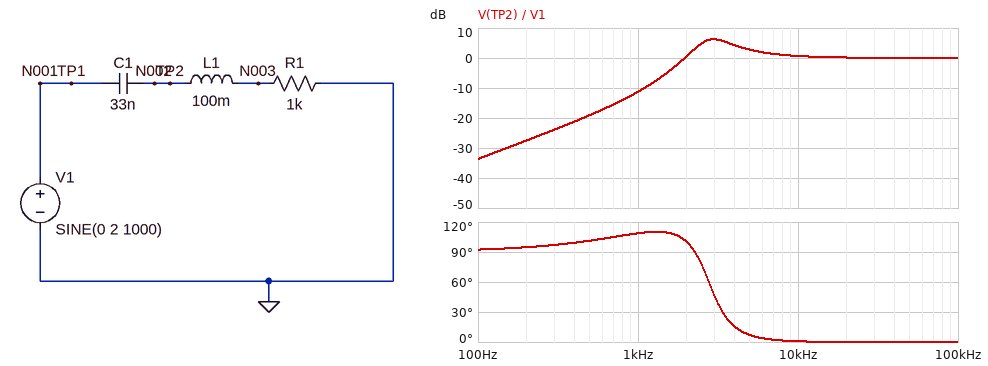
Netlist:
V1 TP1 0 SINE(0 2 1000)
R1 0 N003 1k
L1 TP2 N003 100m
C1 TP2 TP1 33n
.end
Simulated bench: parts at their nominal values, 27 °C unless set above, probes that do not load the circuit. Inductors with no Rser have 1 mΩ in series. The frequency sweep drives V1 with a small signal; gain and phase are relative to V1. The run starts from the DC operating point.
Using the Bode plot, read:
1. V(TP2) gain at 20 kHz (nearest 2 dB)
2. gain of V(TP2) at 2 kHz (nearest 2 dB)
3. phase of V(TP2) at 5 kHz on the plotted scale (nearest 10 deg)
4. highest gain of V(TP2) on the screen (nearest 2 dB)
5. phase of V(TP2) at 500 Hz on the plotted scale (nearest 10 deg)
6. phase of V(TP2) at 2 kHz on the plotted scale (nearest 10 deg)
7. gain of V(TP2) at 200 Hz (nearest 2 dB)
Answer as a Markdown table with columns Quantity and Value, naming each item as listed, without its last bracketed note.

| Quantity | Value |
|---|---|
| V(TP2) gain at 20 kHz | 0 dB |
| gain of V(TP2) at 2 kHz | 0 dB |
| phase of V(TP2) at 5 kHz on the plotted scale | 10 deg |
| highest gain of V(TP2) on the screen | 6 dB |
| phase of V(TP2) at 500 Hz on the plotted scale | 100 deg |
| phase of V(TP2) at 2 kHz on the plotted scale | 100 deg |
| gain of V(TP2) at 200 Hz | -28 dB |
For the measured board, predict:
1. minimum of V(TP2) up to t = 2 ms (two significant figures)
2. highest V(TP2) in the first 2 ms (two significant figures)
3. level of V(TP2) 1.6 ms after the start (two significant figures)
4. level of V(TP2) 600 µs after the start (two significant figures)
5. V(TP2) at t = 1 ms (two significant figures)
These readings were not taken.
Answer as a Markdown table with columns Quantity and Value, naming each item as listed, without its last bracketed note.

| Quantity | Value |
|---|---|
| minimum of V(TP2) up to t = 2 ms | -580 mV |
| highest V(TP2) in the first 2 ms | 750 mV |
| level of V(TP2) 1.6 ms after the start | -320 mV |
| level of V(TP2) 600 µs after the start | -310 mV |
| V(TP2) at t = 1 ms | 520 mV |
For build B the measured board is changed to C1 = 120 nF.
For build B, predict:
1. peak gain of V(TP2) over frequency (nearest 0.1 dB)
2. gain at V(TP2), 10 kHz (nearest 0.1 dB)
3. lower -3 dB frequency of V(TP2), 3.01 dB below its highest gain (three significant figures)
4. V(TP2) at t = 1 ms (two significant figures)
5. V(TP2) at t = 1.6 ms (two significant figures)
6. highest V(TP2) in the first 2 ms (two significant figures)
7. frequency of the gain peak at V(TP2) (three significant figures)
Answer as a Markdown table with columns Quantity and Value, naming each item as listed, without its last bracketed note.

| Quantity | Value |
|---|---|
| peak gain of V(TP2) over frequency | 3.0 dB |
| gain at V(TP2), 10 kHz | 0.2 dB |
| lower -3 dB frequency of V(TP2), 3.01 dB below its highest gain | 1.02 kHz |
| V(TP2) at t = 1 ms | 1.8 V |
| V(TP2) at t = 1.6 ms | -1.9 V |
| highest V(TP2) in the first 2 ms | 1.9 V |
| frequency of the gain peak at V(TP2) | 1.73 kHz |
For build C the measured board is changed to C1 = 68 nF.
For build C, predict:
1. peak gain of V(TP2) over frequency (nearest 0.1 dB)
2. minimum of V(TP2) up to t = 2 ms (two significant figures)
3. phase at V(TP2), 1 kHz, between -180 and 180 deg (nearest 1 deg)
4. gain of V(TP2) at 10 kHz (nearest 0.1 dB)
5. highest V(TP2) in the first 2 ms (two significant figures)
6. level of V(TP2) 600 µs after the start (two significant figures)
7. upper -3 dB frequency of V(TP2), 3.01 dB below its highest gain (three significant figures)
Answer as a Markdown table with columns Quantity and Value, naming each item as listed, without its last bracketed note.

| Quantity | Value |
|---|---|
| peak gain of V(TP2) over frequency | 4.2 dB |
| minimum of V(TP2) up to t = 2 ms | -1.3 V |
| phase at V(TP2), 1 kHz, between -180 and 180 deg | 92 deg |
| gain of V(TP2) at 10 kHz | 0.3 dB |
| highest V(TP2) in the first 2 ms | 1.2 V |
| level of V(TP2) 600 µs after the start | -990 mV |
| upper -3 dB frequency of V(TP2), 3.01 dB below its highest gain | 5.08 kHz |
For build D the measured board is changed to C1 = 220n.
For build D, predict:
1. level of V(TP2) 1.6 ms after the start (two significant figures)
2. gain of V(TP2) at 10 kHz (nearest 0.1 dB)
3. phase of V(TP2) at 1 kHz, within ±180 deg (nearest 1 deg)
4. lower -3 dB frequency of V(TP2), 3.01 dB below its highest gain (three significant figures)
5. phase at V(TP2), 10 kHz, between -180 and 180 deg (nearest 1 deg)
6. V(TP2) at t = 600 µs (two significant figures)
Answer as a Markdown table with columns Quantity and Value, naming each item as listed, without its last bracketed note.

| Quantity | Value |
|---|---|
| level of V(TP2) 1.6 ms after the start | -2.3 V |
| gain of V(TP2) at 10 kHz | 0.1 dB |
| phase of V(TP2) at 1 kHz, within ±180 deg | 38 deg |
| lower -3 dB frequency of V(TP2), 3.01 dB below its highest gain | 652 Hz |
| phase at V(TP2), 10 kHz, between -180 and 180 deg | 0 deg |
| V(TP2) at t = 600 µs | -2.2 V |
